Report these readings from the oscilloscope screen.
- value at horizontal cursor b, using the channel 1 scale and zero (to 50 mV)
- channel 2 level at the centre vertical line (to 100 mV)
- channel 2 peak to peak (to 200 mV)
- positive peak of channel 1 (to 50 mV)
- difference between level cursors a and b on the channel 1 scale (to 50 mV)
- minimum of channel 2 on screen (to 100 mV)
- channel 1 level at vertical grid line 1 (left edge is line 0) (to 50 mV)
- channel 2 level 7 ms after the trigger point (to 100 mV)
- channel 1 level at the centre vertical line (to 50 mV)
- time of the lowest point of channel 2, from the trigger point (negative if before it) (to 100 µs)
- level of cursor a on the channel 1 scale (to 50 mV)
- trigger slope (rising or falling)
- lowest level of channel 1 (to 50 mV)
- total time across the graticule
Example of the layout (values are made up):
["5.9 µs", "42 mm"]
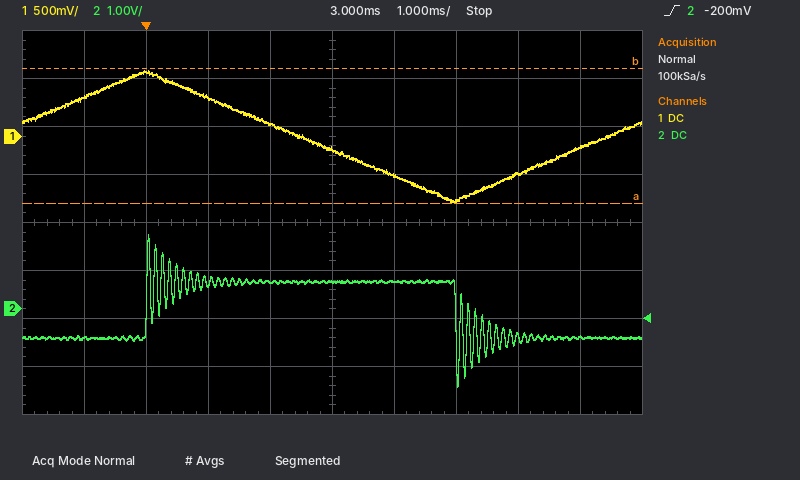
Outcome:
["700 mV", "600 mV", "3.2 V", "700 mV", "1.40 V", "-1.6 V", "400 mV", "-600 mV", "-150 mV", "+5.0 ms", "-700 mV", "rising", "-700 mV", "10 ms"]
